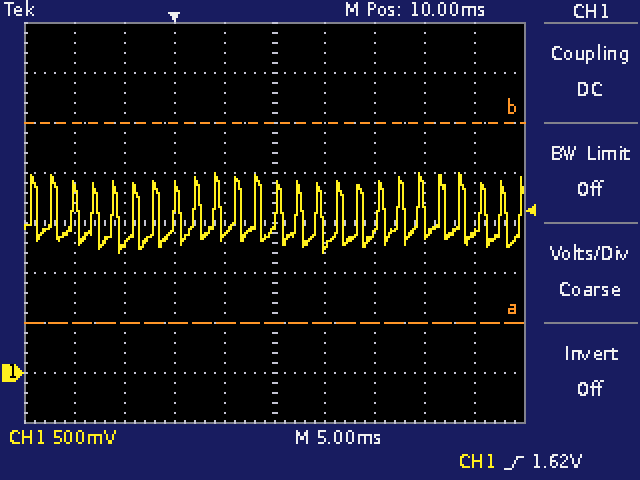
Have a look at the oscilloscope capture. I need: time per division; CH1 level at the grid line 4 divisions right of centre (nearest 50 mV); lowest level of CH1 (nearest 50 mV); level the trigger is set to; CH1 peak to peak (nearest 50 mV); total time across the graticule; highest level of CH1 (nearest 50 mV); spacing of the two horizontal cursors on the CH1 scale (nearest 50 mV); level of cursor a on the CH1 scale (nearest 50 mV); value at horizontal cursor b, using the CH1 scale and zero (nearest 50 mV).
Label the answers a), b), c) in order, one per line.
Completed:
a) 5 ms
b) 1.40 V
c) 1.20 V
d) 1.62 V
e) 800 mV
f) 50 ms
g) 2.00 V
h) 2.00 V
i) 500 mV
j) 2.50 V
